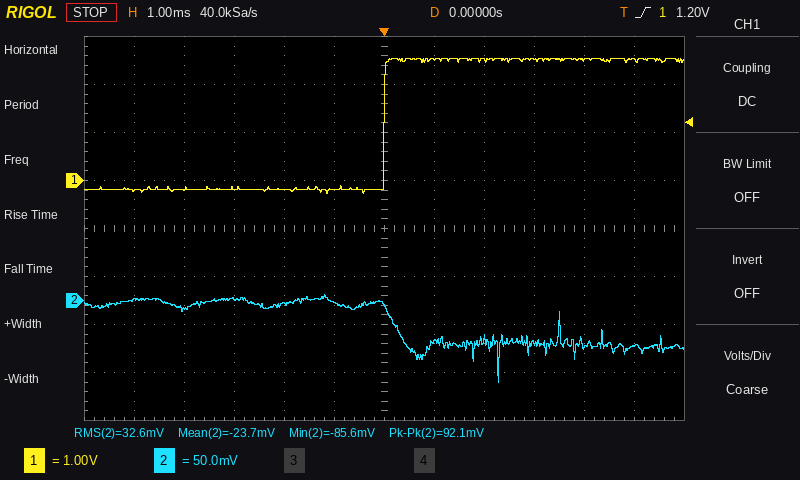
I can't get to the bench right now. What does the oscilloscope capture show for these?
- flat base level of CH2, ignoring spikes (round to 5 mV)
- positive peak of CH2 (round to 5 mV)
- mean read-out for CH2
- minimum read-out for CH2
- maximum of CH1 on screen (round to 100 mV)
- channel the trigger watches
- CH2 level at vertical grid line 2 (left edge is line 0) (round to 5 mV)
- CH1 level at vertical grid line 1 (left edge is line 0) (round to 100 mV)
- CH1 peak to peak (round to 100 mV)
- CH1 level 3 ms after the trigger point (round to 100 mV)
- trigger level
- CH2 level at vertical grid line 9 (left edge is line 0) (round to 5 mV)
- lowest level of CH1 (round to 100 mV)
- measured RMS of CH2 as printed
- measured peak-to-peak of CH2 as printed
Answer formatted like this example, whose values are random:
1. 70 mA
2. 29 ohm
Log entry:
1. -45 mV
2. 5 mV
3. -23.7 mV
4. -85.6 mV
5. 2.5 V
6. CH1
7. -10 mV
8. -200 mV
9. 2.8 V
10. 2.5 V
11. 1.20 V
12. -45 mV
13. -300 mV
14. 32.6 mV
15. 92.1 mV
